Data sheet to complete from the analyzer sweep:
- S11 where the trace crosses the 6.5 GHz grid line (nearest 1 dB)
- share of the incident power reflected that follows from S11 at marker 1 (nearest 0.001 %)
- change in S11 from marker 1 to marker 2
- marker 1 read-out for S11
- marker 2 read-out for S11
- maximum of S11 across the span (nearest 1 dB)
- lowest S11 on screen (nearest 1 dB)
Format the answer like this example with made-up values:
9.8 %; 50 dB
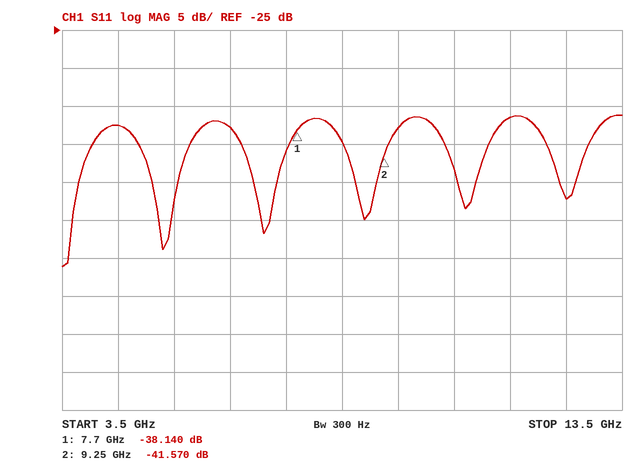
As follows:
-38 dB; 0.015 %; -3.430 dB; -38.140 dB; -41.570 dB; -36 dB; -56 dB
